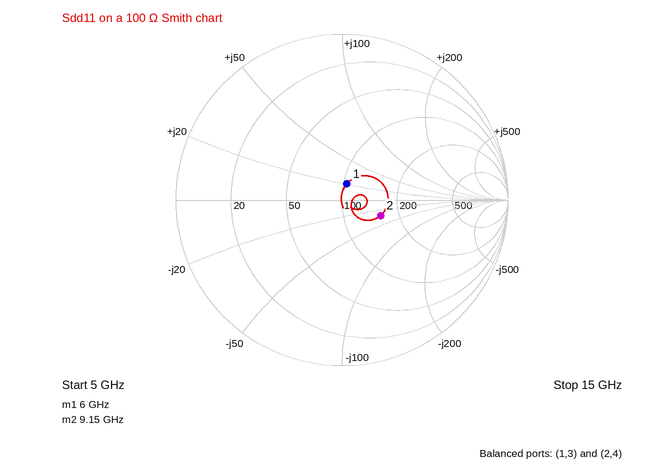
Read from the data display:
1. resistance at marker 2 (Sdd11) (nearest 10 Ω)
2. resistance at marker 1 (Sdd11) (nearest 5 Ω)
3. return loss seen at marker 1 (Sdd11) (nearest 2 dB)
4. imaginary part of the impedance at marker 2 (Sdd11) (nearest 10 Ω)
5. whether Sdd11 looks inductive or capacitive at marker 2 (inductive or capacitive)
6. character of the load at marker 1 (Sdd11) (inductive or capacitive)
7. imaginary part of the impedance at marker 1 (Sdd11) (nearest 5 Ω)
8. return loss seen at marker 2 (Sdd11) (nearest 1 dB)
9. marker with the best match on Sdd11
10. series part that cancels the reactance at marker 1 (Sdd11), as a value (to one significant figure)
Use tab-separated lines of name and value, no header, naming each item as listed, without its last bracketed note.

resistance at marker 2 (Sdd11)	160 Ω
resistance at marker 1 (Sdd11)	105 Ω
return loss seen at marker 1 (Sdd11)	20 dB
imaginary part of the impedance at marker 2 (Sdd11)	-30 Ω
whether Sdd11 looks inductive or capacitive at marker 2	capacitive
character of the load at marker 1 (Sdd11)	inductive
imaginary part of the impedance at marker 1 (Sdd11)	+20 Ω
return loss seen at marker 2 (Sdd11)	12 dB
marker with the best match on Sdd11	marker 1
series part that cancels the reactance at marker 1 (Sdd11), as a value	1 pF
